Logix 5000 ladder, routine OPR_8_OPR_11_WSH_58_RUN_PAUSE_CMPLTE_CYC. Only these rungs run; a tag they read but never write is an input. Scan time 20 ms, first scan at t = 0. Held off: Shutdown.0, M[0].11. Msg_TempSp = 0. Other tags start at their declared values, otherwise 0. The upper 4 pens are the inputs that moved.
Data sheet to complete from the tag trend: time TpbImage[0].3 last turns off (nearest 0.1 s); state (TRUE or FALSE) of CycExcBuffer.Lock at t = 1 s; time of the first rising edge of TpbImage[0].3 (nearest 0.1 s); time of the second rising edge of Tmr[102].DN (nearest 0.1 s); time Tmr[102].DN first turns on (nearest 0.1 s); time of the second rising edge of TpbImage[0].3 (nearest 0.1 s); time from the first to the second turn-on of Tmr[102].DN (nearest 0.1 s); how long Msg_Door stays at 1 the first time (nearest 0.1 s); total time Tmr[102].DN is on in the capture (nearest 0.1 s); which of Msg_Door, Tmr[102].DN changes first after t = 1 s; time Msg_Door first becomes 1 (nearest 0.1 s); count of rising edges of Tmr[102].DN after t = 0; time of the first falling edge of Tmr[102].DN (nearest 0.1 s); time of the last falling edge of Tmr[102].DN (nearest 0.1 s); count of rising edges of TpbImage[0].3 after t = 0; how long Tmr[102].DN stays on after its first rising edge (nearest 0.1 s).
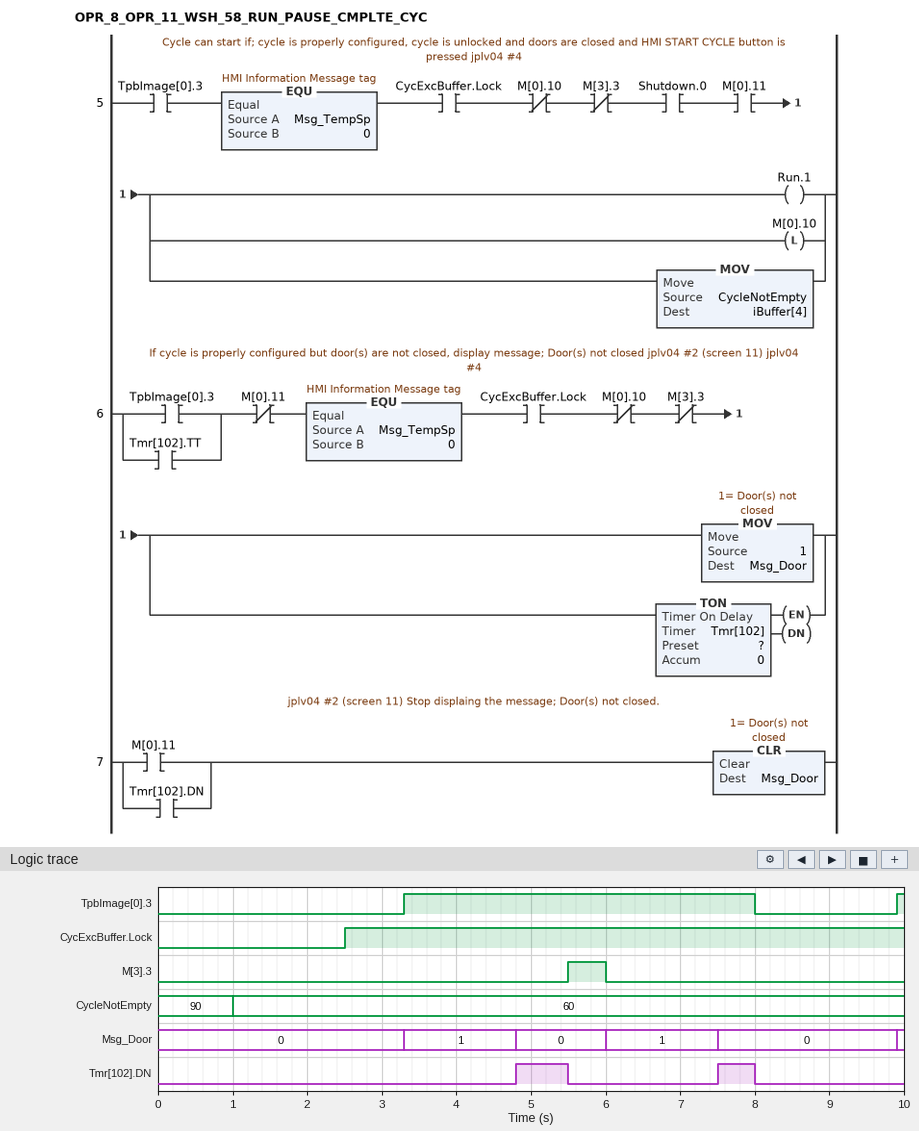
8.0 s
FALSE
3.3 s
7.5 s
4.8 s
9.9 s
2.7 s
1.5 s
1.2 s
Msg_Door
3.3 s
2
5.5 s
8.0 s
2
0.7 s
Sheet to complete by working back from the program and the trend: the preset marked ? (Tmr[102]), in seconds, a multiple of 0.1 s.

1.5 s
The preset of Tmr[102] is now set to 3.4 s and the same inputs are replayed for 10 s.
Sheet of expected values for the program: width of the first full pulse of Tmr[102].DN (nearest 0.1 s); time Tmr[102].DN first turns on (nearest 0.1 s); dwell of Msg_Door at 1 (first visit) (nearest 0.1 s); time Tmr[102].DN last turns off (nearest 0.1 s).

0.0 s
9.4 s
6.1 s
9.4 s
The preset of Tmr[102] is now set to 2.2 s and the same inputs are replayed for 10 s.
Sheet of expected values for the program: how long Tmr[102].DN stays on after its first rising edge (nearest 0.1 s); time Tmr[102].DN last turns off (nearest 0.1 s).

0.0 s
8.2 s
